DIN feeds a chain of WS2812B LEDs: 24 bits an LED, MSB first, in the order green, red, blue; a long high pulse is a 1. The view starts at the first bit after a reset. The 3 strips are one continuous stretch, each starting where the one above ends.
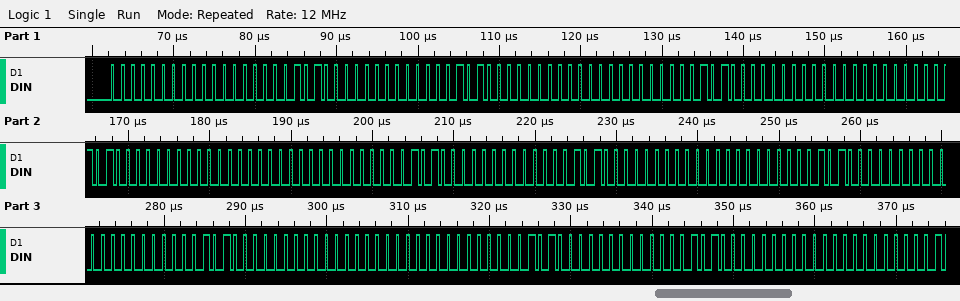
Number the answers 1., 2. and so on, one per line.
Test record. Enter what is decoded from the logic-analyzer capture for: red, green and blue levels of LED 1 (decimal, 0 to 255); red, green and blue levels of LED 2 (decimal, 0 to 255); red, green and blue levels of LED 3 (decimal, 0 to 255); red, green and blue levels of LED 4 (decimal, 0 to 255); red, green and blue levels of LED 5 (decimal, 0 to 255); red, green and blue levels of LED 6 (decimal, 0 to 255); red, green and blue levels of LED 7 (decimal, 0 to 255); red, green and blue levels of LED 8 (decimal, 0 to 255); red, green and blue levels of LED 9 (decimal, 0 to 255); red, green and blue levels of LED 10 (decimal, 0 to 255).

1. 0, 0, 40
2. 40, 0, 0
3. 40, 0, 0
4. 40, 0, 0
5. 0, 0, 40
6. 40, 0, 0
7. 40, 0, 0
8. 40, 0, 0
9. 0, 0, 40
10. 40, 0, 0
